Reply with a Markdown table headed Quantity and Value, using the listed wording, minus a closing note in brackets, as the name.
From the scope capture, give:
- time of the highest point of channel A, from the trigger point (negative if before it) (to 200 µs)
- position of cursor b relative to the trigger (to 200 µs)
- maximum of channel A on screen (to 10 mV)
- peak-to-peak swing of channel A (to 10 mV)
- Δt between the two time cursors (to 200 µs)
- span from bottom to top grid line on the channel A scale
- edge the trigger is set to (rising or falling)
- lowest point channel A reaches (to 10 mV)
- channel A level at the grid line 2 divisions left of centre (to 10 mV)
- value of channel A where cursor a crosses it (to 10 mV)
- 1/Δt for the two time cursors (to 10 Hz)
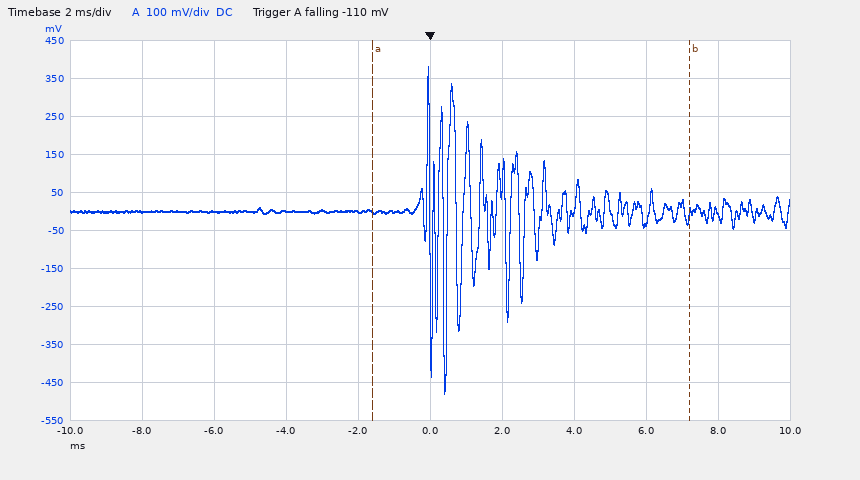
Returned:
| Quantity | Value |
|---|---|
| time of the highest point of channel A, from the trigger point (negative if before it) | 0.0 ms |
| position of cursor b relative to the trigger | +7.2 ms |
| maximum of channel A on screen | 380 mV |
| peak-to-peak swing of channel A | 860 mV |
| Δt between the two time cursors | 8.8 ms |
| span from bottom to top grid line on the channel A scale | 1 V |
| edge the trigger is set to | falling |
| lowest point channel A reaches | -480 mV |
| channel A level at the grid line 2 divisions left of centre | 0 mV |
| value of channel A where cursor a crosses it | 0 mV |
| 1/Δt for the two time cursors | 110 Hz |
